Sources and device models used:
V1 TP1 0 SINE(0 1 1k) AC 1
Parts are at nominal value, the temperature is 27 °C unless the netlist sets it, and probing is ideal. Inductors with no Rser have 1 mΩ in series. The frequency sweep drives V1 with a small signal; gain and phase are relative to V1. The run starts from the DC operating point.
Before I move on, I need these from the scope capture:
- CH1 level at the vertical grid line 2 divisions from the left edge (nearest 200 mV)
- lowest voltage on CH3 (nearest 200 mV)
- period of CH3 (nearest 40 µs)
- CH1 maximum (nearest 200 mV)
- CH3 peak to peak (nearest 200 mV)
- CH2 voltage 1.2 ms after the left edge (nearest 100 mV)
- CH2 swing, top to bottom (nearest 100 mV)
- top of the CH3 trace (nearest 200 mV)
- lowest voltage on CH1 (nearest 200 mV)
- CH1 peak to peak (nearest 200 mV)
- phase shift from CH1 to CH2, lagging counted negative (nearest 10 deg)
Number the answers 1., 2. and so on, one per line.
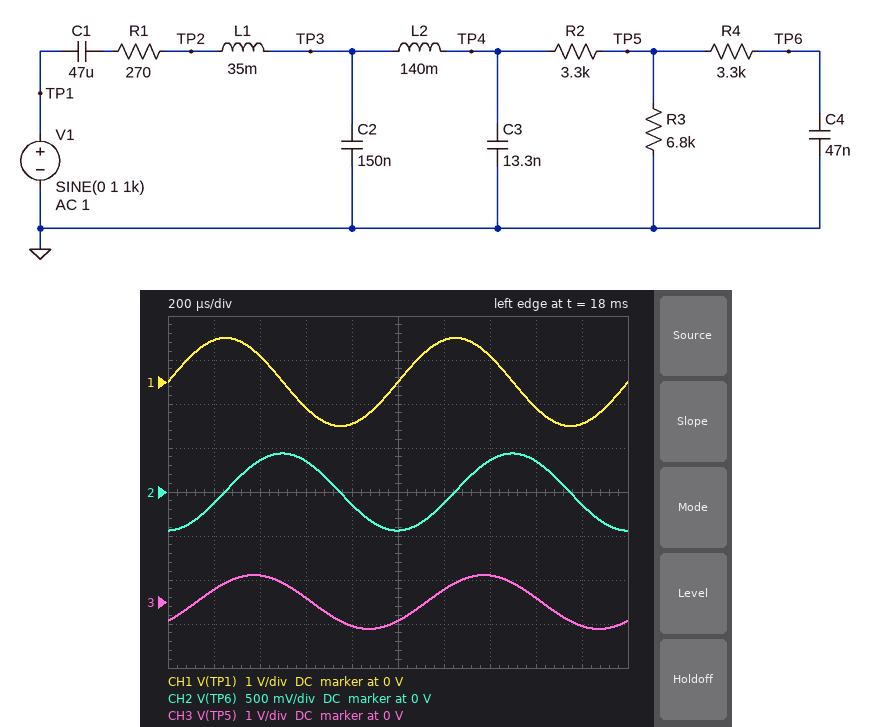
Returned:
1. 600 mV
2. -600 mV
3. 1.00 ms
4. 1.0 V
5. 1.2 V
6. -100 mV
7. 900 mV
8. 600 mV
9. -1.0 V
10. 2.0 V
11. -90 deg
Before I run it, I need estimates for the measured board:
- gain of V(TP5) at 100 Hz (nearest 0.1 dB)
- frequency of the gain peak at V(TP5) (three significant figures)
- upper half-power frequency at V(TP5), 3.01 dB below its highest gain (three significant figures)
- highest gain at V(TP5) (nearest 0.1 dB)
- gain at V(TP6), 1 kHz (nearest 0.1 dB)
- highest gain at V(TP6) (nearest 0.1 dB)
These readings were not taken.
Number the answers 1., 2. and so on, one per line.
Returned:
1. -3.7 dB
2. 1.99 kHz
3. 2.92 kHz
4. -1.7 dB
5. -7.2 dB
6. -3.7 dB
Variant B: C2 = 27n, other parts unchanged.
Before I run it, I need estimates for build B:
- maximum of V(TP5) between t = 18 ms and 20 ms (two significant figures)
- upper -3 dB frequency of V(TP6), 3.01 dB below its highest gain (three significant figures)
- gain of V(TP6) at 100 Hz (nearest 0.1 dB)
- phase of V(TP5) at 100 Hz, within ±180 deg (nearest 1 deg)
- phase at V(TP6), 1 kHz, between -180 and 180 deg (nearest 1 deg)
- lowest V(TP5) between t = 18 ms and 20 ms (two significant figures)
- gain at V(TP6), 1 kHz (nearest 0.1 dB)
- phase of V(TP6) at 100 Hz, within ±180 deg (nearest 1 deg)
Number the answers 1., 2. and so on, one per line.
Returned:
1. 540 mV
2. 700 Hz
3. -3.8 dB
4. -5 deg
5. -74 deg
6. -540 mV
7. -8.2 dB
8. -10 deg
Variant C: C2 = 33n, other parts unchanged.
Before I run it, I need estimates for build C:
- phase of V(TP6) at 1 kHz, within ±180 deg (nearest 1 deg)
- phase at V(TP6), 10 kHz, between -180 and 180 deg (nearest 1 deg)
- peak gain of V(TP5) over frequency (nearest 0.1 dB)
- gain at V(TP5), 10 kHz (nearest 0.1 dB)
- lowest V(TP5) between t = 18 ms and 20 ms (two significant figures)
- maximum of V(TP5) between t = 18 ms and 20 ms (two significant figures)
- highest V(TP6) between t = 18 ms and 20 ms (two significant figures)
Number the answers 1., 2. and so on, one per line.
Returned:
1. -75 deg
2. -63 deg
3. -1.3 dB
4. -34.7 dB
5. -550 mV
6. 550 mV
7. 390 mV
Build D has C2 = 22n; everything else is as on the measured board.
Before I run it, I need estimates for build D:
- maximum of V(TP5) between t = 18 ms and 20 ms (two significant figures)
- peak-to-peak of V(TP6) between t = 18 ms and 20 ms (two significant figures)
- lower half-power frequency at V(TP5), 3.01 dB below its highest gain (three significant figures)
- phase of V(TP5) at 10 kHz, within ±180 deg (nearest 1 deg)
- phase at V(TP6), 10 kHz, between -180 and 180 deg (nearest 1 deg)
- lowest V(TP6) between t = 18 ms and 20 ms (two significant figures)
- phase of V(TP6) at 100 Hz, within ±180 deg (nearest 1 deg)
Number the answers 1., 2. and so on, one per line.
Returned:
1. 540 mV
2. 770 mV
3. 434 mHz
4. 23 deg
5. -61 deg
6. -390 mV
7. -10 deg
